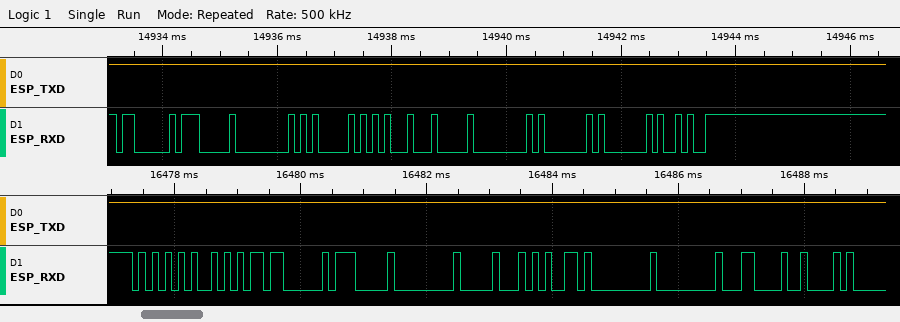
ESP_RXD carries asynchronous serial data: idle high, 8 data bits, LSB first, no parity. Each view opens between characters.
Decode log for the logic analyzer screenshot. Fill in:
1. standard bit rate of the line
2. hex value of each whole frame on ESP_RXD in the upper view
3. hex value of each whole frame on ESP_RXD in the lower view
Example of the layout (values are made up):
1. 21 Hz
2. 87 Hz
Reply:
1. 9600 baud
2. 03, 07, 00, 05, 15, 04, 00, 01, 01, 29
3. 55, AA, 03, 07, 00, 10, 65, 00, 00, 0C, 42
